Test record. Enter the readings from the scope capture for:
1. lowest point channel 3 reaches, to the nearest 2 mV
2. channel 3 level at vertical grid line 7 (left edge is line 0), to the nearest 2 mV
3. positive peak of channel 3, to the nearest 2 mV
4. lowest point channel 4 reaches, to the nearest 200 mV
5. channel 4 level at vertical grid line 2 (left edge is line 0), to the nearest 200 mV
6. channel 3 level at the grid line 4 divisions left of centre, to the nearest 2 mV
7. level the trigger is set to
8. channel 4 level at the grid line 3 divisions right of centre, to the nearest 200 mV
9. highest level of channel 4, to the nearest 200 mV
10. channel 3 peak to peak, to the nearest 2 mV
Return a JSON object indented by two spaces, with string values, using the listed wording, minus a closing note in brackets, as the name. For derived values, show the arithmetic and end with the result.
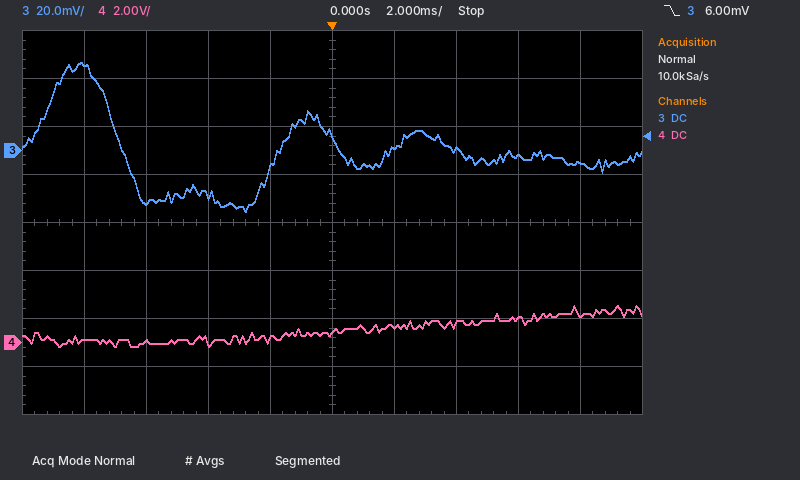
{
  "lowest point channel 3 reaches, to the nearest 2 mV": "-26 mV",
  "channel 3 level at vertical grid line 7 (left edge is line 0), to the nearest 2 mV": "0 mV",
  "positive peak of channel 3, to the nearest 2 mV": "36 mV",
  "lowest point channel 4 reaches, to the nearest 200 mV": "-200 mV",
  "channel 4 level at vertical grid line 2 (left edge is line 0), to the nearest 200 mV": "0.0 V",
  "channel 3 level at the grid line 4 divisions left of centre, to the nearest 2 mV": "36 mV",
  "level the trigger is set to": "6.00 mV",
  "channel 4 level at the grid line 3 divisions right of centre, to the nearest 200 mV": "1.0 V",
  "highest level of channel 4, to the nearest 200 mV": "1.6 V",
  "channel 3 peak to peak, to the nearest 2 mV": "36 mV − (-26 mV) = 62 mV"
}
